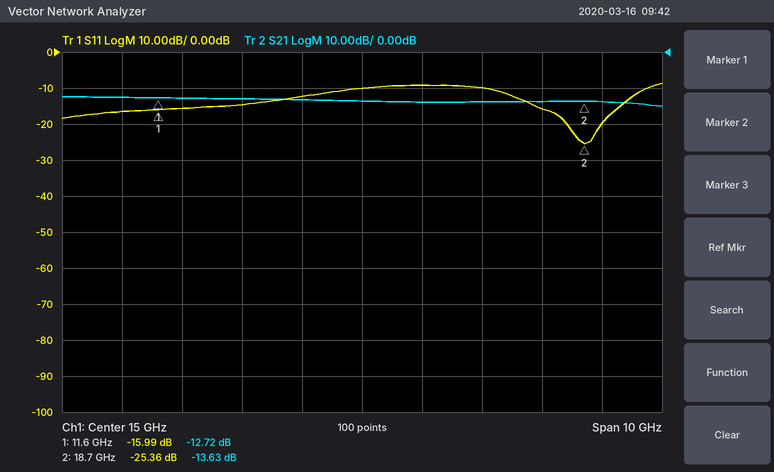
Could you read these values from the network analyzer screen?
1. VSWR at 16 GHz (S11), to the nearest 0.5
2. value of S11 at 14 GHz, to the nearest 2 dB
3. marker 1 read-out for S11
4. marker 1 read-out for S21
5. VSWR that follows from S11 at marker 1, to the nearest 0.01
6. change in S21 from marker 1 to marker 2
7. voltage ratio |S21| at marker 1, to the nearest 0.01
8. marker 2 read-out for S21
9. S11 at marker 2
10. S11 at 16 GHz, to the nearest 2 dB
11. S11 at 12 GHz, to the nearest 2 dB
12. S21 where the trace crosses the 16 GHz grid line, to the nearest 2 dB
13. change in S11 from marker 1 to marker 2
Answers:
2.0
-12 dB
-15.99 dB
-12.72 dB
1.38
-0.91 dB
0.23
-13.63 dB
-25.36 dB
-10 dB
-16 dB
-14 dB
-9.37 dB
